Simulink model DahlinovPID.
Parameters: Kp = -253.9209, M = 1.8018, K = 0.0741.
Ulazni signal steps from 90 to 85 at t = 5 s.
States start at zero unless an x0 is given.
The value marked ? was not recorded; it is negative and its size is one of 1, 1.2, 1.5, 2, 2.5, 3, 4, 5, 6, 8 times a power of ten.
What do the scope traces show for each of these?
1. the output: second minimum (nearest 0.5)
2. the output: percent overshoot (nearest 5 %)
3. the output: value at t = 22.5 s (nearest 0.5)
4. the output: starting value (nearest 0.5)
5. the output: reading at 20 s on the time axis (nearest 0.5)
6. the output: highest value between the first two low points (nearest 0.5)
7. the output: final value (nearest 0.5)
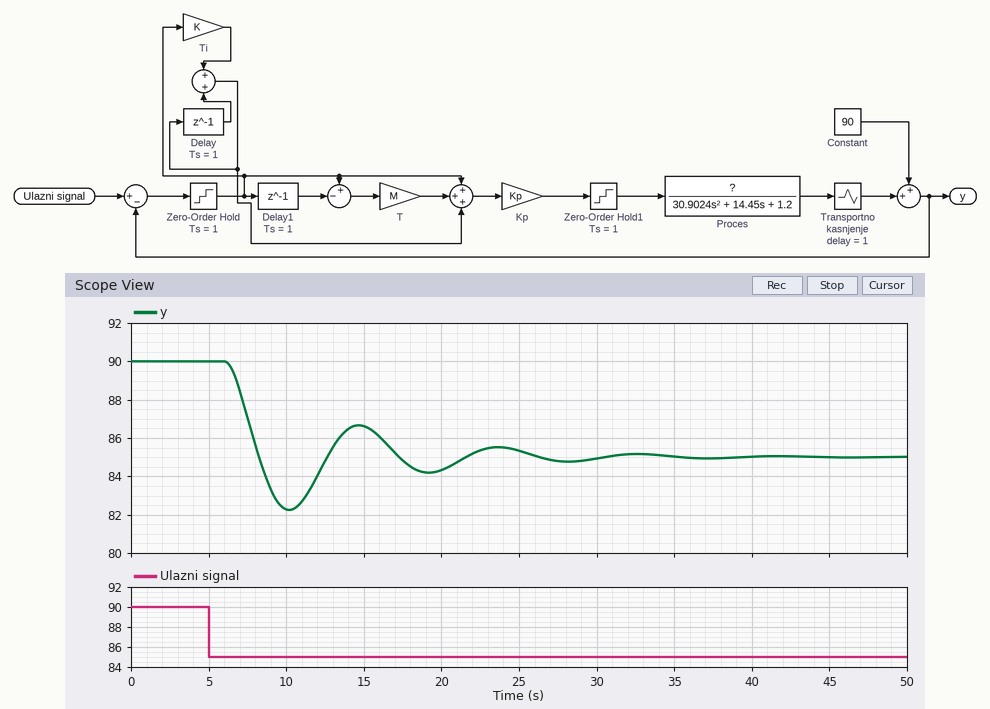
84.0
55 %
85.5
90.0
84.5
86.5
85.0
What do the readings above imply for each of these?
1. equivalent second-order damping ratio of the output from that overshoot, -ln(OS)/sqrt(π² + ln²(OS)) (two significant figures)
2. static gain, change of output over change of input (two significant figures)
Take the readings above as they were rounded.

0.19
1.0
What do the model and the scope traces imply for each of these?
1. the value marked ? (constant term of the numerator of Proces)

-0.03
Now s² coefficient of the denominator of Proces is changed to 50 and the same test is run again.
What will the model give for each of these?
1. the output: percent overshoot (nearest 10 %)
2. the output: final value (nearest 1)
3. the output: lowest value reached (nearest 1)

50 %
85
82
